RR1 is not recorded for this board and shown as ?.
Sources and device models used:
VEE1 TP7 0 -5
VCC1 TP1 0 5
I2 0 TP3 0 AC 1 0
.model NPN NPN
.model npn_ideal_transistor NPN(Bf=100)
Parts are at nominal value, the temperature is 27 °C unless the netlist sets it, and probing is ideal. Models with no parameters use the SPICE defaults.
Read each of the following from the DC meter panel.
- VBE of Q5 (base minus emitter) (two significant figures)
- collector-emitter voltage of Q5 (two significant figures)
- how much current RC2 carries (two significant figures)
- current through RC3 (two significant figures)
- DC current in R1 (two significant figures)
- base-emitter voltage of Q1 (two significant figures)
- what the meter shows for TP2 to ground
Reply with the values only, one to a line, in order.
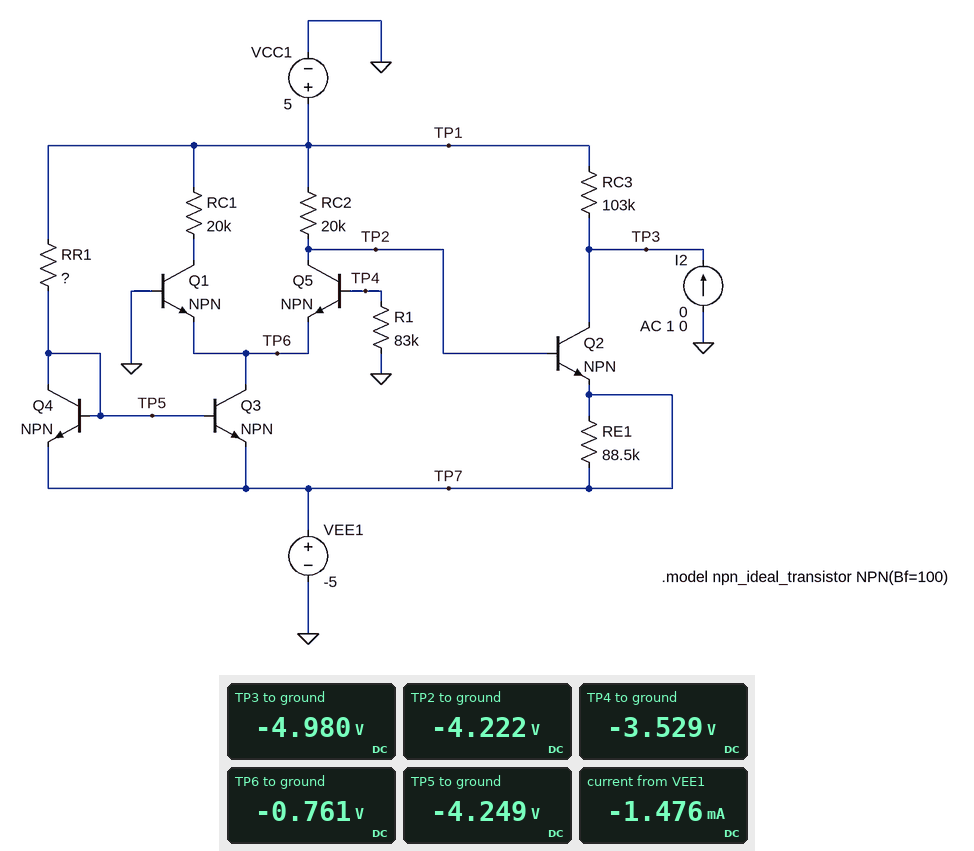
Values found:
-2.8 V
-3.5 V
460 µA
97 µA
43 µA
760 mV
-4.222 V
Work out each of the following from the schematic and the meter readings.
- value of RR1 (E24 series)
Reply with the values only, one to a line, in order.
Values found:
22 kΩ
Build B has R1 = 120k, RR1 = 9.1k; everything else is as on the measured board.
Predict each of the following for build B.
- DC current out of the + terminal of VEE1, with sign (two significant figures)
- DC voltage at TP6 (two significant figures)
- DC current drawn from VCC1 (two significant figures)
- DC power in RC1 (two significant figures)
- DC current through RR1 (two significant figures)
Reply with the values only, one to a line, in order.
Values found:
-2.6 mA
-790 mV
1.9 mA
1.7 mW
1.0 mA
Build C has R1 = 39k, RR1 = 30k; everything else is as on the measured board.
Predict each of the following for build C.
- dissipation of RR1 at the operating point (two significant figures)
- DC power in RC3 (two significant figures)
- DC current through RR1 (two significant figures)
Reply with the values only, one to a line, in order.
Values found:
2.9 mW
970 µW
310 µA
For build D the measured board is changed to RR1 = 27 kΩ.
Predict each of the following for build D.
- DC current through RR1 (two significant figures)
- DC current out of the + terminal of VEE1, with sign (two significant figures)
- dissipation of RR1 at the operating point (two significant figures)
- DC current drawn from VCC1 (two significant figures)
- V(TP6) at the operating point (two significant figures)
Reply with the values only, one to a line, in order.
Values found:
340 µA
-1.3 mA
3.2 mW
1.2 mA
-750 mV
